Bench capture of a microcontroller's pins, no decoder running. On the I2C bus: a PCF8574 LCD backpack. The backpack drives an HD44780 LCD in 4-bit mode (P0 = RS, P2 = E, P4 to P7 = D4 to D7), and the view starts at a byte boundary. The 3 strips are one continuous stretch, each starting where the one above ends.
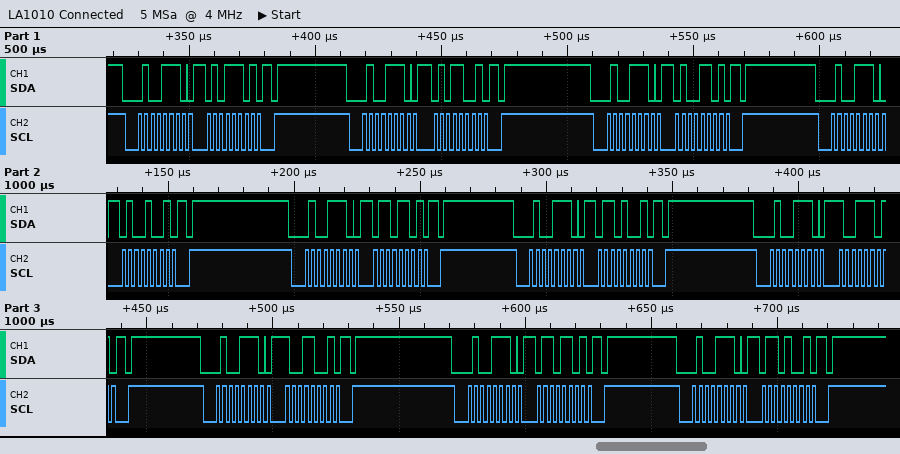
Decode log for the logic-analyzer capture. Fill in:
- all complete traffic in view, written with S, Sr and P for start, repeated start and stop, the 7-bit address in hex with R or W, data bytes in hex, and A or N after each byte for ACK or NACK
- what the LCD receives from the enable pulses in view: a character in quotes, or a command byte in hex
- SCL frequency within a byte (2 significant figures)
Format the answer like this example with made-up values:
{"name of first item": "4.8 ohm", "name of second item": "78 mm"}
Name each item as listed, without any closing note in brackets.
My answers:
{"all complete traffic in view, written with S, Sr and P for start, repeated start and stop, the 7-bit address in hex with R or W, data bytes in hex, and A or N after each byte for ACK or NACK": "S 27W A 5D A P S 27W A 59 A P S 27W A 4D A P S 27W A 49 A P S 27W A 6D A P S 27W A 69 A P S 27W A 9D A P S 27W A 99 A P S 27W A 6D A P S 27W A 69 A P", "what the LCD receives from the enable pulses in view: a character in quotes, or a command byte in hex": "'T' 'i'", "SCL frequency within a byte": "400 kHz"}
